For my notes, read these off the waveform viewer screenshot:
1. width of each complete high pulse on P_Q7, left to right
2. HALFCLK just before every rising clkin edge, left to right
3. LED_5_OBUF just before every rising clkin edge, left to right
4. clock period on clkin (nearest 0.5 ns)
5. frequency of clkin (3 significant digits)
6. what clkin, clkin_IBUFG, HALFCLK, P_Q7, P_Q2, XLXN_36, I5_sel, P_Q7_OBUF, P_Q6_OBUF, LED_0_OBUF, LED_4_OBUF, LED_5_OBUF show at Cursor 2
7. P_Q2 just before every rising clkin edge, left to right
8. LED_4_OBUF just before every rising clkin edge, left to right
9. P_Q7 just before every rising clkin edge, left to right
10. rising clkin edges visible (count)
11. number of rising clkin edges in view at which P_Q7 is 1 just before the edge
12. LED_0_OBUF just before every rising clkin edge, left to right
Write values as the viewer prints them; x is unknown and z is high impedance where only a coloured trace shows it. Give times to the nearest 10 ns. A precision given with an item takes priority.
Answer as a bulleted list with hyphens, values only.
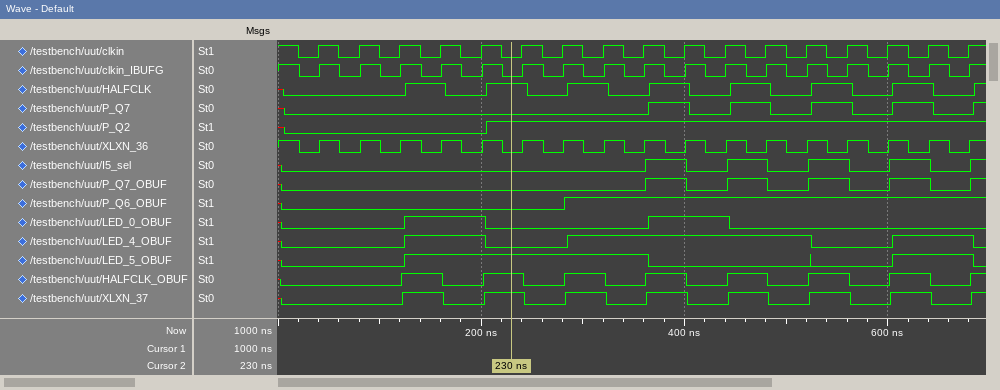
- 40 ns, 40 ns, 40 ns, 40 ns
- 0 0 0 1 0 1 0 1 0 1 0 1 0 1 0 1 0
- 0 0 0 1 1 1 1 1 1 0 0 0 0 0 0 1 1
- 40 ns
- 25.0 MHz
- clkin=0, clkin_IBUFG=0, HALFCLK=1, P_Q7=0, P_Q2=1, XLXN_36=0, I5_sel=0, P_Q7_OBUF=0, P_Q6_OBUF=0, LED_0_OBUF=0, LED_4_OBUF=0, LED_5_OBUF=1
- 0 0 0 0 0 1 1 1 1 1 1 1 1 1 1 1 1
- 0 0 0 1 1 0 0 1 1 1 1 1 1 0 0 1 1
- 0 0 0 0 0 0 0 0 0 1 0 1 0 1 0 1 0
- 17
- 4
- 0 0 0 1 1 0 0 0 0 1 1 0 0 0 0 0 0
